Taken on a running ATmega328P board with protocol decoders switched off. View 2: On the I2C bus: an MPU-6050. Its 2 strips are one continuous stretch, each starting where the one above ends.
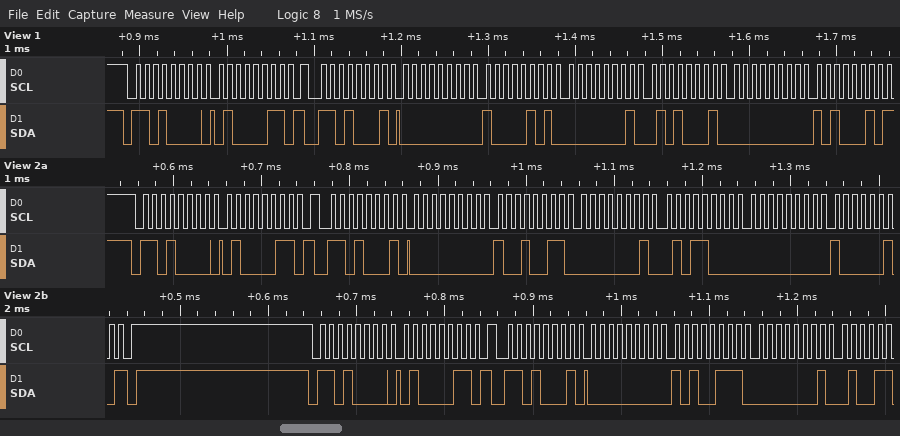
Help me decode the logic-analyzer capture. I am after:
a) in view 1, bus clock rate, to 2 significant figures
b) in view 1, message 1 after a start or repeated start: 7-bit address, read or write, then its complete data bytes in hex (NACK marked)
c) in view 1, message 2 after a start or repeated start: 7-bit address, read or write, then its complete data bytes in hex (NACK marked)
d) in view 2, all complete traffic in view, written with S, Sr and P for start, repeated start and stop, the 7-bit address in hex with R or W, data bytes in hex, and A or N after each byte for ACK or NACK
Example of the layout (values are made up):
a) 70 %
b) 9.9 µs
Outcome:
a) 100 kHz
b) 0x68 write: 43
c) 0x68 read: 00 85 01 51 00 A2 NACK
d) S 68W A 43 A Sr 68R A 00 A 93 A 01 A 58 A 00 A 82 N P S 68W A 43 A Sr 68R A 00 A A7 A 01 A
